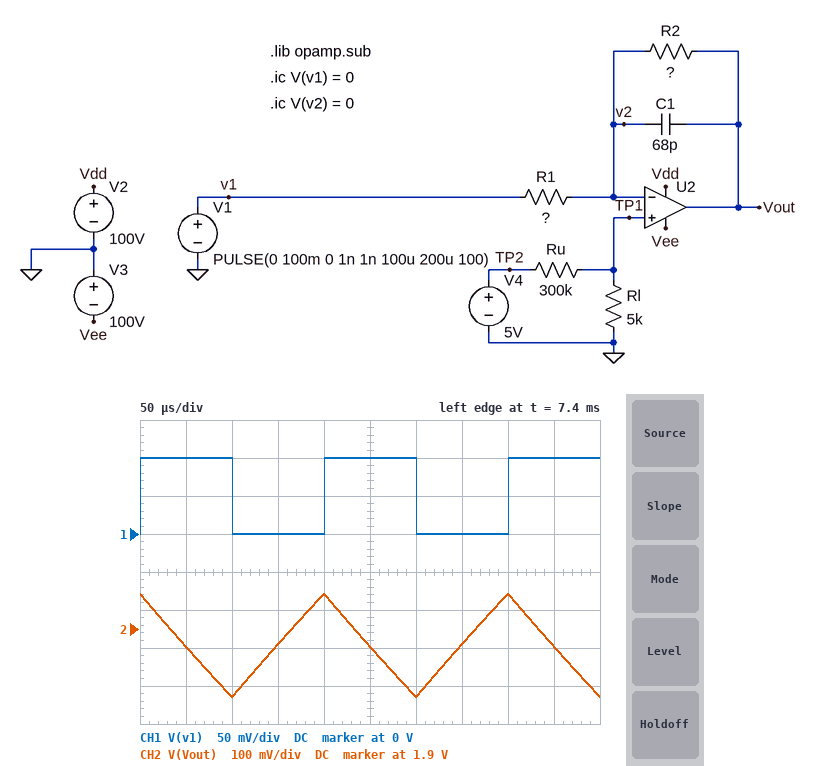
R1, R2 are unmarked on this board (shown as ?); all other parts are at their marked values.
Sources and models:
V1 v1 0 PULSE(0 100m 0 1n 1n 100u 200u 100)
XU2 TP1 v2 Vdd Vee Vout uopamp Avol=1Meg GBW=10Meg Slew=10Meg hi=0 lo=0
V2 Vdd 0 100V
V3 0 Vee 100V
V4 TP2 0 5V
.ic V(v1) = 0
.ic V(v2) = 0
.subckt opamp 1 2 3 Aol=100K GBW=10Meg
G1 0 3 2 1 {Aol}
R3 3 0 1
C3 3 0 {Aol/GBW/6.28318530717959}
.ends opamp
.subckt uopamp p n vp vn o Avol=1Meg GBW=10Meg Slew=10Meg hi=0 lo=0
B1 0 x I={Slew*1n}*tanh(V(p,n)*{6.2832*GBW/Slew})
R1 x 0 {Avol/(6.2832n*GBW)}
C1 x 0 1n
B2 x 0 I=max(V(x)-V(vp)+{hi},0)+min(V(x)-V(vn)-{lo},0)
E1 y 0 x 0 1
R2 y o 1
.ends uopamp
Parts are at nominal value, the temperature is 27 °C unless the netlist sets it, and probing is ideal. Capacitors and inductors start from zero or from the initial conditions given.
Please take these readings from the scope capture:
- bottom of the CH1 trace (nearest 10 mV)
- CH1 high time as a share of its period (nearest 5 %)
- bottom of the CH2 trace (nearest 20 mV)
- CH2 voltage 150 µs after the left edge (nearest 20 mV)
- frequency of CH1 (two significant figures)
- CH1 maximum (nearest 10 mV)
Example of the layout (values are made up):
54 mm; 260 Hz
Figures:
0 V; 50 %; 1.72 V; 1.86 V; 5.0 kHz; 100 mV
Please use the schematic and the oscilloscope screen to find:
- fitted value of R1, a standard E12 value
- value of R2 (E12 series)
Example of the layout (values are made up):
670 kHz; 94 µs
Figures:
270 kΩ; 15 MΩ
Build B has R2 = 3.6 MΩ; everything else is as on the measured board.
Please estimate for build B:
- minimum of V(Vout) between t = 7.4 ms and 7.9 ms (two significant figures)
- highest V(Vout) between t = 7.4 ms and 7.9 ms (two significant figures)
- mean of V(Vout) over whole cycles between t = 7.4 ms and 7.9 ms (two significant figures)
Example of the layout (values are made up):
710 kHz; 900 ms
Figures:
370 mV; 640 mV; 510 mV
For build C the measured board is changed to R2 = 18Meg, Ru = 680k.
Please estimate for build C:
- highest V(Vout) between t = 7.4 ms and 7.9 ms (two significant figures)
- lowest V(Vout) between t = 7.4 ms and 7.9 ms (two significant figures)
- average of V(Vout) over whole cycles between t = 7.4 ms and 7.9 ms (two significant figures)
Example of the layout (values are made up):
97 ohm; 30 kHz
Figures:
-730 mV; -1.0 V; -860 mV
